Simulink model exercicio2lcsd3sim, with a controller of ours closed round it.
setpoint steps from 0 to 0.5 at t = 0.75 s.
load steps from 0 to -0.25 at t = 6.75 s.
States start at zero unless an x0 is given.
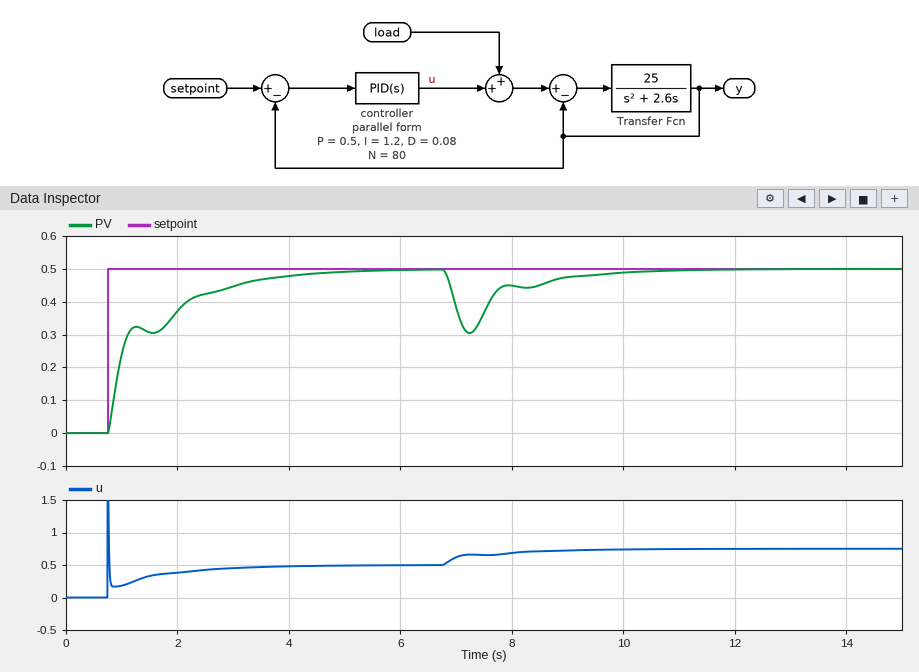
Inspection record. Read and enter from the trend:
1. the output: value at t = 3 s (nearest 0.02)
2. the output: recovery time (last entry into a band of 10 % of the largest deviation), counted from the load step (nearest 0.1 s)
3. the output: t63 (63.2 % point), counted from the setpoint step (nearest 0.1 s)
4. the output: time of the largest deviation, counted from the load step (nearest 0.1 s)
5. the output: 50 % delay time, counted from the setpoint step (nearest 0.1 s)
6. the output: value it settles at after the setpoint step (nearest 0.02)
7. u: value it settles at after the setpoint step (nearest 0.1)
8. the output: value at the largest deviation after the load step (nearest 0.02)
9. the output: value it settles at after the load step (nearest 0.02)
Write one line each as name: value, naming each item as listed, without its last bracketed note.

the output: value at t = 3 s: 0.44
the output: recovery time (last entry into a band of 10 % of the largest deviation), counted from the load step: 2.7 s
the output: t63 (63.2 % point), counted from the setpoint step: 0.4 s
the output: time of the largest deviation, counted from the load step: 0.5 s
the output: 50 % delay time, counted from the setpoint step: 0.3 s
the output: value it settles at after the setpoint step: 0.50
u: value it settles at after the setpoint step: 0.5
the output: value at the largest deviation after the load step: 0.30
the output: value it settles at after the load step: 0.50
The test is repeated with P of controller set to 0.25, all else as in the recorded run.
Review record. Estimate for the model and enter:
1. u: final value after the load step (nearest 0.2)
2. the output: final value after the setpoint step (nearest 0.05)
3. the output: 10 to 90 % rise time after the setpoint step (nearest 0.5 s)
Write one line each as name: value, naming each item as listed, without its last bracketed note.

u: final value after the load step: 0.8
the output: final value after the setpoint step: 0.50
the output: 10 to 90 % rise time after the setpoint step: 2.0 s
